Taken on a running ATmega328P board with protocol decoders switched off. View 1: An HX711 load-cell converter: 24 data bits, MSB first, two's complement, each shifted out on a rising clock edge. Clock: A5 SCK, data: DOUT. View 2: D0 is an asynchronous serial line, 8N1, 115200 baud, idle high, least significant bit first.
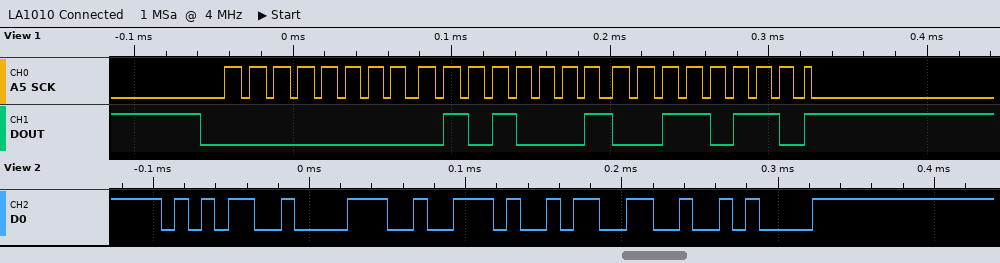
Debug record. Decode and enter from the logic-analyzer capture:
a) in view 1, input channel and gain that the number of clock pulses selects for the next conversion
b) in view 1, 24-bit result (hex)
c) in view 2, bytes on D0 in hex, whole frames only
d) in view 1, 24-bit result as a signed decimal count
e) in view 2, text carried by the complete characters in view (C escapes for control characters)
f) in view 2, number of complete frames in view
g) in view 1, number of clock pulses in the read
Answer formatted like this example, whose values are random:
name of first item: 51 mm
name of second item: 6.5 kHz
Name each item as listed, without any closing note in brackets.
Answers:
in view 1, input channel and gain that the number of clock pulses selects for the next conversion: channel A, gain 128
in view 1, 24-bit result: 0x005136
in view 2, bytes on D0 in hex, whole frames only: 35 38 2E 33 0A
in view 1, 24-bit result as a signed decimal count: 20790
in view 2, text carried by the complete characters in view: "58.3\n"
in view 2, number of complete frames in view: 5
in view 1, number of clock pulses in the read: 25
